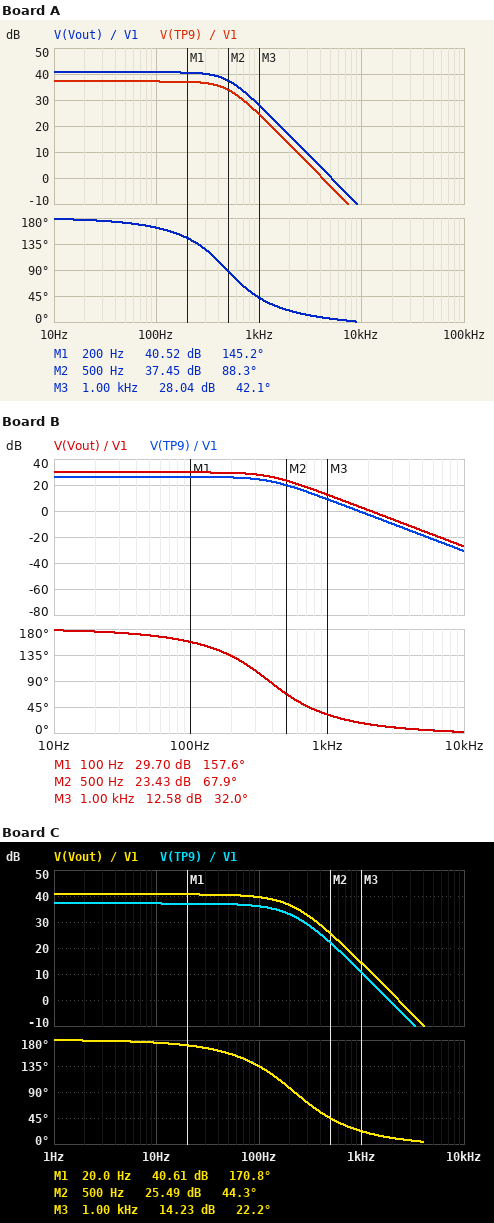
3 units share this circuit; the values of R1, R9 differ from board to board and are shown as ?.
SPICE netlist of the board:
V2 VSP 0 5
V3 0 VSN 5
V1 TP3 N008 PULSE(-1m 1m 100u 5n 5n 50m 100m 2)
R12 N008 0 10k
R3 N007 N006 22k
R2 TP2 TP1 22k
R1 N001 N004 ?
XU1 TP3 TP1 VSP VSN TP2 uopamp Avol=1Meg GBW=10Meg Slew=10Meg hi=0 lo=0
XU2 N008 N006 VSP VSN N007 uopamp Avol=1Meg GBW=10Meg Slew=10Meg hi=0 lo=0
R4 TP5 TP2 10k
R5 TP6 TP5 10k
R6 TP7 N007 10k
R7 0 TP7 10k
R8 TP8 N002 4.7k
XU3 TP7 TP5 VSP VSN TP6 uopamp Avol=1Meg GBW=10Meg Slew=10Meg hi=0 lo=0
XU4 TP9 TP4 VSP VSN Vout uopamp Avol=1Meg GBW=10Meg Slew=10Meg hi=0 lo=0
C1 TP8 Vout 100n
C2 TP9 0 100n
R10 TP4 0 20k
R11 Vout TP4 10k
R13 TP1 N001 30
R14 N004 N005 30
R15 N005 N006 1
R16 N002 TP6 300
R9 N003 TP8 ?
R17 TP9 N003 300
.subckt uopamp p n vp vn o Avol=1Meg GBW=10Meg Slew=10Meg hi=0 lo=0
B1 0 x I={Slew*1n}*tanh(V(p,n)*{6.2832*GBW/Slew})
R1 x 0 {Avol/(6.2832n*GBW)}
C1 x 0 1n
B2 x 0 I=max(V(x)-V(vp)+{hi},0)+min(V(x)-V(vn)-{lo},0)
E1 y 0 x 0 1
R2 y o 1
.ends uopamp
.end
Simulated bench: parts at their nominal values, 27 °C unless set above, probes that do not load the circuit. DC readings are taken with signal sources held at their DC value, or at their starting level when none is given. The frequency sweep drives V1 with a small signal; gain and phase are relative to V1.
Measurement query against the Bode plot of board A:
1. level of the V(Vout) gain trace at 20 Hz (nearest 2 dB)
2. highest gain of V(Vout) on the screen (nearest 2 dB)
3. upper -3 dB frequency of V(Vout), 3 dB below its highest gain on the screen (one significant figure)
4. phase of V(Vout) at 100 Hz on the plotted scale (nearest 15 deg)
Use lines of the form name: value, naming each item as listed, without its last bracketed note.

level of the V(Vout) gain trace at 20 Hz: 40 dB
highest gain of V(Vout) on the screen: 40 dB
upper -3 dB frequency of V(Vout), 3 dB below its highest gain on the screen: 500 Hz
phase of V(Vout) at 100 Hz on the plotted scale: 165 deg
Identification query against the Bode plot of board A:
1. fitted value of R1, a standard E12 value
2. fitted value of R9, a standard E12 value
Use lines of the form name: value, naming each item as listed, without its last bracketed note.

fitted value of R1, a standard E12 value: 560 Ω
fitted value of R9, a standard E12 value: 1.8 kΩ
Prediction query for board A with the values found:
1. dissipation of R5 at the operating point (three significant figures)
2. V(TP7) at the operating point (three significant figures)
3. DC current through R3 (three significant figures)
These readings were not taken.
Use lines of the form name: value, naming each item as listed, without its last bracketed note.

dissipation of R5 at the operating point: 293 nW
V(TP7) at the operating point: 17.7 mV
DC current through R3: 1.61 µA
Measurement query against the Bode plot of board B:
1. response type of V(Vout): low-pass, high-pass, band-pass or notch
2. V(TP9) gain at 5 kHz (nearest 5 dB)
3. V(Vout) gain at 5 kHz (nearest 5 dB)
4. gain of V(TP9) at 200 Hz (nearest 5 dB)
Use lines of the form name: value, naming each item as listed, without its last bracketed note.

response type of V(Vout): low-pass, high-pass, band-pass or notch: low-pass
V(TP9) gain at 5 kHz: -20 dB
V(Vout) gain at 5 kHz: -15 dB
gain of V(TP9) at 200 Hz: 25 dB
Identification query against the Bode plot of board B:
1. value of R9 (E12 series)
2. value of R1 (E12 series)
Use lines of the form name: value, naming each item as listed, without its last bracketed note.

value of R9: 3.3 kΩ
value of R1: 2.2 kΩ
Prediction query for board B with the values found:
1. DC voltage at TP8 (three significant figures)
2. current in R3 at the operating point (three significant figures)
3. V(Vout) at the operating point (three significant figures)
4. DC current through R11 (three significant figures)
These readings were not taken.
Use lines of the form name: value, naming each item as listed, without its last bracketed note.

DC voltage at TP8: 20.5 mV
current in R3 at the operating point: 442 nA
V(Vout) at the operating point: 30.7 mV
DC current through R11: 1.02 µA
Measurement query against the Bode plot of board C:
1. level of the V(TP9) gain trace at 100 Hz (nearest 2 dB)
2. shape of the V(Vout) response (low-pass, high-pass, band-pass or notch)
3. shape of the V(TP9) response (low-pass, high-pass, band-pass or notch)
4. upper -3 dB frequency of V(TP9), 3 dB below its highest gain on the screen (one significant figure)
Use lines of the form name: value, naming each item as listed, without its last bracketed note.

level of the V(TP9) gain trace at 100 Hz: 36 dB
shape of the V(Vout) response: low-pass
shape of the V(TP9) response: low-pass
upper -3 dB frequency of V(TP9), 3 dB below its highest gain on the screen: 200 Hz
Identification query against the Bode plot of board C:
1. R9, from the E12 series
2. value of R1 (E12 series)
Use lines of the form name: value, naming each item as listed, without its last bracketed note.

R9, from the E12 series: 10 kΩ
value of R1: 560 Ω
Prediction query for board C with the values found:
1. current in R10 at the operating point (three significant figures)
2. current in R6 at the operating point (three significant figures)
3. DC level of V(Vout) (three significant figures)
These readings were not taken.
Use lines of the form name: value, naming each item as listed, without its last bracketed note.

current in R10 at the operating point: 3.59 µA
current in R6 at the operating point: 1.77 µA
DC level of V(Vout): 108 mV
